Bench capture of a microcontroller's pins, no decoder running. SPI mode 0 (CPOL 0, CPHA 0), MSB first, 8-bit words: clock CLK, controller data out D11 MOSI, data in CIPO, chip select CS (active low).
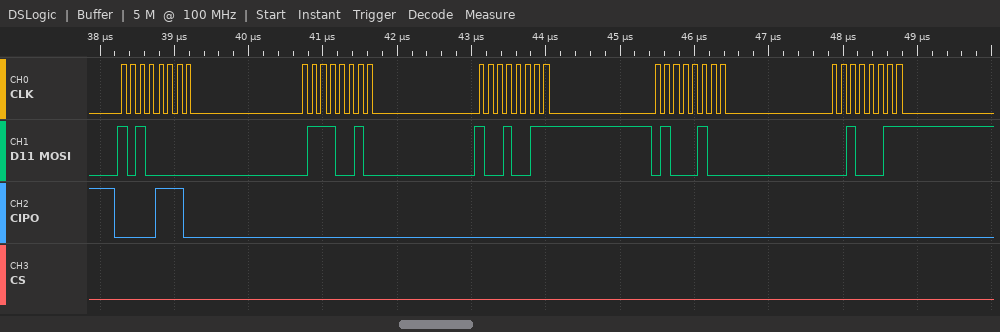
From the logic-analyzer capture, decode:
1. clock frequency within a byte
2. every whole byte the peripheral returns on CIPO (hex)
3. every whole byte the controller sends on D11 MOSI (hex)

8 MHz
0E 00 00 00 00
A0 72 93 44 23
